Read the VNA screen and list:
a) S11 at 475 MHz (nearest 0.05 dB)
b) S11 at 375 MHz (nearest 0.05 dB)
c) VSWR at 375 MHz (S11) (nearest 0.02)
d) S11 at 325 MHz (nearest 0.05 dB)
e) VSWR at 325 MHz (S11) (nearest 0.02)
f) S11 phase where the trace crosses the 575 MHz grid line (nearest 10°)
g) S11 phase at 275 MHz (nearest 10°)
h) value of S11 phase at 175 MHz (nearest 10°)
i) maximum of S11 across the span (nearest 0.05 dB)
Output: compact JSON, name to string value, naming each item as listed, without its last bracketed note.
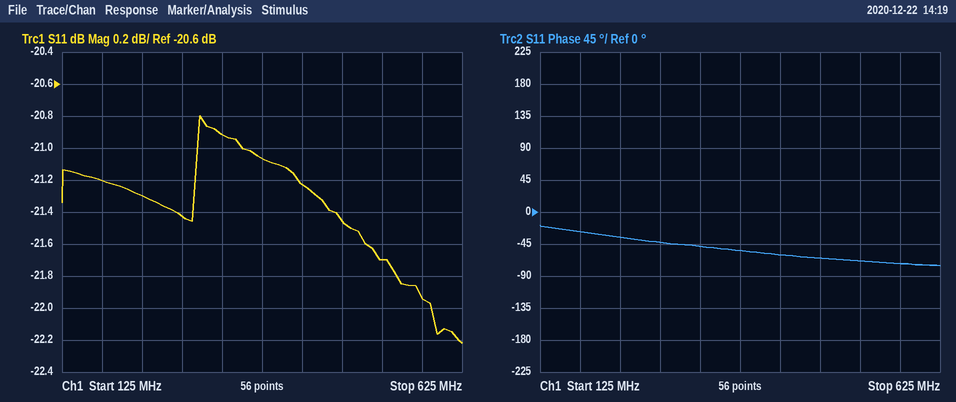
{"S11 at 475 MHz": "-21.45 dB", "S11 at 375 MHz": "-21.05 dB", "VSWR at 375 MHz (S11)": "1.20", "S11 at 325 MHz": "-20.90 dB", "VSWR at 325 MHz (S11)": "1.20", "S11 phase where the trace crosses the 575 MHz grid line": "-70°", "S11 phase at 275 MHz": "-40°", "value of S11 phase at 175 MHz": "-30°", "maximum of S11 across the span": "-20.80 dB"}
